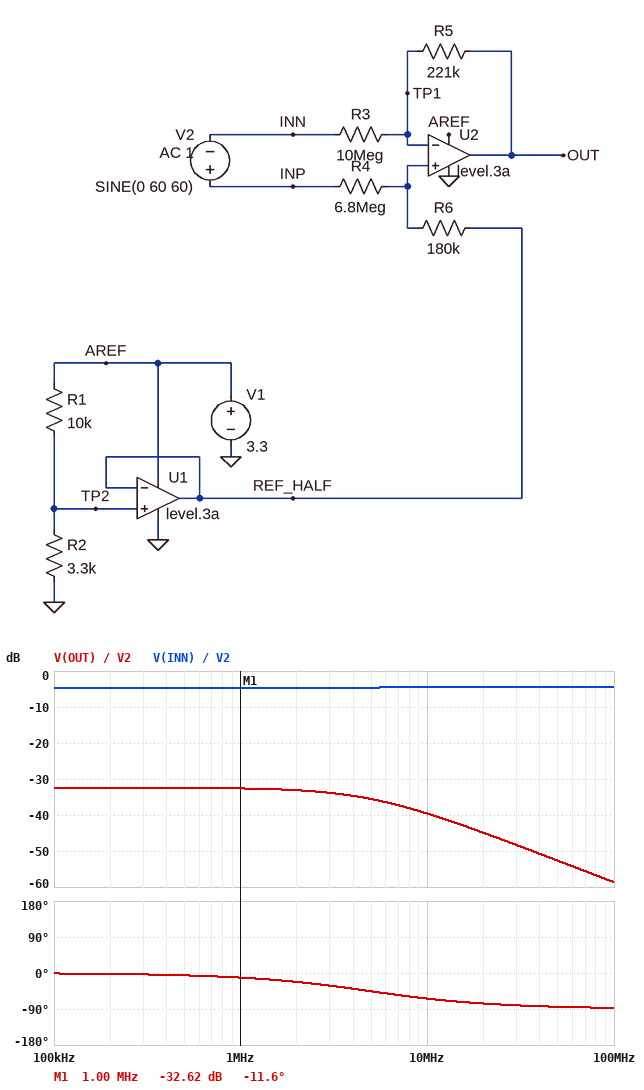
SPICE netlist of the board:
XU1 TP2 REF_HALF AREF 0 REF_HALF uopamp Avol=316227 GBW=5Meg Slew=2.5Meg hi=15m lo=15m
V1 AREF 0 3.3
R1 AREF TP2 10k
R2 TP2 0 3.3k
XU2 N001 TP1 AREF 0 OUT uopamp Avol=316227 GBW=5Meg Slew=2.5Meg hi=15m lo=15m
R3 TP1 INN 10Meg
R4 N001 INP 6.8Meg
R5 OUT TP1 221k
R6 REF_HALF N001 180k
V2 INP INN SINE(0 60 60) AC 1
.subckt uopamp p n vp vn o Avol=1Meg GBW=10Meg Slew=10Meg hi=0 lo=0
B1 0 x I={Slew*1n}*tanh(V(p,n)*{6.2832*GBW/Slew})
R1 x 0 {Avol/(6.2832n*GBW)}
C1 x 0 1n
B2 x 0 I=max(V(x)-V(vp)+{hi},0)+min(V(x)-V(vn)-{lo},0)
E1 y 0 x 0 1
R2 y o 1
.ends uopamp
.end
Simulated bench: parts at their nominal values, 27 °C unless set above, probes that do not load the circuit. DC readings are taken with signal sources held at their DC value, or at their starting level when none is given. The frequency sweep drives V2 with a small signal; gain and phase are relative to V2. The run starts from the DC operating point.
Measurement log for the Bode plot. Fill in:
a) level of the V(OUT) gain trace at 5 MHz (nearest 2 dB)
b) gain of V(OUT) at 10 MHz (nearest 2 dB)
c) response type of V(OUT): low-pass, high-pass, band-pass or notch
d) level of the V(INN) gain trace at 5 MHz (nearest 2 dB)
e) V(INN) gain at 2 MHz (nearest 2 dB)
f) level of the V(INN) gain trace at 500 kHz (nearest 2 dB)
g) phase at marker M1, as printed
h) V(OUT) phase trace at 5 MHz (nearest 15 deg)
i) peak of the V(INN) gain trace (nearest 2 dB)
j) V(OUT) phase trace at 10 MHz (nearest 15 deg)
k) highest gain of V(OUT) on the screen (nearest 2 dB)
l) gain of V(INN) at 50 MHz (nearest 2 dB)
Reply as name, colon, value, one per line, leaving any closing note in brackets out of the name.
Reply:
level of the V(OUT) gain trace at 5 MHz: -36 dB
gain of V(OUT) at 10 MHz: -40 dB
response type of V(OUT): low-pass, high-pass, band-pass or notch: low-pass
level of the V(INN) gain trace at 5 MHz: -4 dB
V(INN) gain at 2 MHz: -4 dB
level of the V(INN) gain trace at 500 kHz: -4 dB
phase at marker M1, as printed: -11.6 deg
V(OUT) phase trace at 5 MHz: -45 deg
peak of the V(INN) gain trace: -4 dB
V(OUT) phase trace at 10 MHz: -60 deg
highest gain of V(OUT) on the screen: -32 dB
gain of V(INN) at 50 MHz: -4 dB
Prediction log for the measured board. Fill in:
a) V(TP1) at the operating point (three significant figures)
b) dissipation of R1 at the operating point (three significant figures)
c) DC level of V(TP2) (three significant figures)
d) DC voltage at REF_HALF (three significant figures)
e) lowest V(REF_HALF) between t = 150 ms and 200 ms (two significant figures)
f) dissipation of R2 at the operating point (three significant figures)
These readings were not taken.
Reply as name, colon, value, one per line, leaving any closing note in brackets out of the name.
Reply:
V(TP1) at the operating point: 819 mV
dissipation of R1 at the operating point: 616 µW
DC level of V(TP2): 819 mV
DC voltage at REF_HALF: 819 mV
lowest V(REF_HALF) between t = 150 ms and 200 ms: 820 mV
dissipation of R2 at the operating point: 203 µW
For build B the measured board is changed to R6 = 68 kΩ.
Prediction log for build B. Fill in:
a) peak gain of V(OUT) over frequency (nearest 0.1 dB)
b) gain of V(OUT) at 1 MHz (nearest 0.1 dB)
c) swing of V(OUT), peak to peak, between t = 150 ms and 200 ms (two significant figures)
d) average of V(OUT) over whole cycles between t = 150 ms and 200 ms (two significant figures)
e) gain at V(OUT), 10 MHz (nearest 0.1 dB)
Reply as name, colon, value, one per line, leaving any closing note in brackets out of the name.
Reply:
peak gain of V(OUT) over frequency: -35.3 dB
gain of V(OUT) at 1 MHz: -35.5 dB
swing of V(OUT), peak to peak, between t = 150 ms and 200 ms: 1.8 V
average of V(OUT) over whole cycles between t = 150 ms and 200 ms: 850 mV
gain at V(OUT), 10 MHz: -42.4 dB
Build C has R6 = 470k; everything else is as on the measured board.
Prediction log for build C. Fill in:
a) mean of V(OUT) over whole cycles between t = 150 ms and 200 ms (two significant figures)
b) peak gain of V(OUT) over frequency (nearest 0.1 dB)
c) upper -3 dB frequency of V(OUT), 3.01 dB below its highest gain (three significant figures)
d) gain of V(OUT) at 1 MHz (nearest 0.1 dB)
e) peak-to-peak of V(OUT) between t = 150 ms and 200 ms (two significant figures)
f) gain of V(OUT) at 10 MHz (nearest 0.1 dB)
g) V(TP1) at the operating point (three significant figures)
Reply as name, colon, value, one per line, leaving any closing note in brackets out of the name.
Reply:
mean of V(OUT) over whole cycles between t = 150 ms and 200 ms: 1.2 V
peak gain of V(OUT) over frequency: -27.7 dB
upper -3 dB frequency of V(OUT), 3.01 dB below its highest gain: 4.80 MHz
gain of V(OUT) at 1 MHz: -27.9 dB
peak-to-peak of V(OUT) between t = 150 ms and 200 ms: 3.3 V
gain of V(OUT) at 10 MHz: -35.0 dB
V(TP1) at the operating point: 819 mV
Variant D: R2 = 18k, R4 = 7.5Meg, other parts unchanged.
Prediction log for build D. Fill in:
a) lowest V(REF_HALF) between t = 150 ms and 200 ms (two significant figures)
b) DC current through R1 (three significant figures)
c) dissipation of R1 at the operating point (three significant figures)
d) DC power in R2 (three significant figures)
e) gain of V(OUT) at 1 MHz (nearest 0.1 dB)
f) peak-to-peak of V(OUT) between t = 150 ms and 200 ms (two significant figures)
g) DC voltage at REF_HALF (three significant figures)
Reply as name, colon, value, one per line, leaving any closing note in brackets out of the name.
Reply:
lowest V(REF_HALF) between t = 150 ms and 200 ms: 2.1 V
DC current through R1: 118 µA
dissipation of R1 at the operating point: 139 µW
DC power in R2: 250 µW
gain of V(OUT) at 1 MHz: -33.0 dB
peak-to-peak of V(OUT) between t = 150 ms and 200 ms: 2.5 V
DC voltage at REF_HALF: 2.12 V
